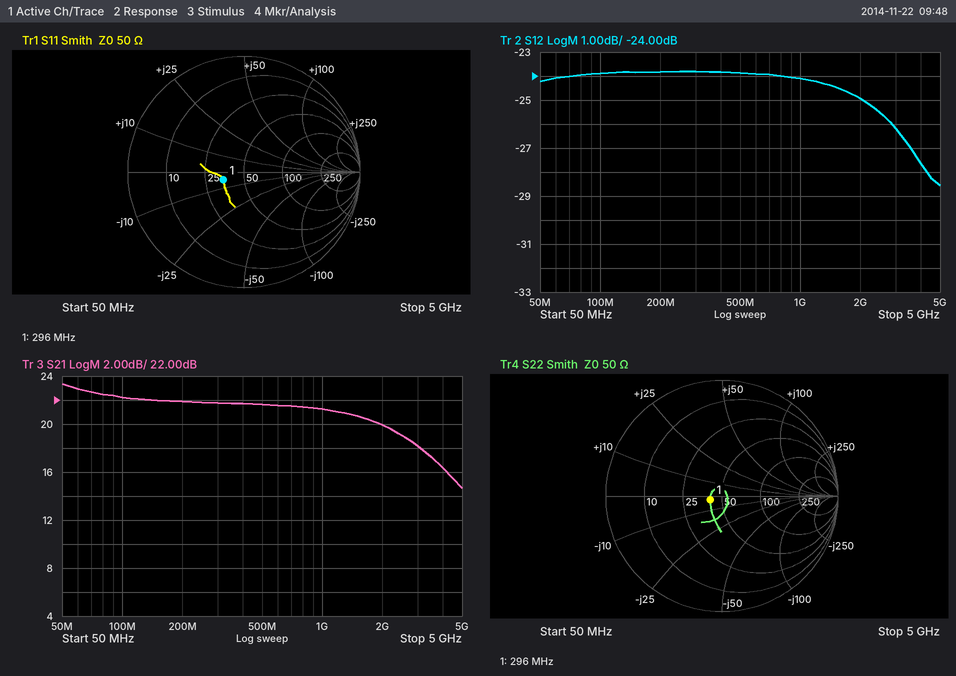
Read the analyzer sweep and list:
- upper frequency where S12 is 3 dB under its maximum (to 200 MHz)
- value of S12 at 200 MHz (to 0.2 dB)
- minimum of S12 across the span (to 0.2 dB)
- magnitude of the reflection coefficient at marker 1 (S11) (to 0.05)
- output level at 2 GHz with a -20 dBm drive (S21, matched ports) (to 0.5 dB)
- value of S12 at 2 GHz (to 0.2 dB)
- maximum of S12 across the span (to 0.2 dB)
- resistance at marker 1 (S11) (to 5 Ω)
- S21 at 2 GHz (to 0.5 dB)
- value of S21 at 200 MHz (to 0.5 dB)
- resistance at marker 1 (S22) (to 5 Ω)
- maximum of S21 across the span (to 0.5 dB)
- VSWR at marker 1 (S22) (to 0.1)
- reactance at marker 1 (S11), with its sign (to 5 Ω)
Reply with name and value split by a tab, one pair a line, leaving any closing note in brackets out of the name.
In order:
upper frequency where S12 is 3 dB under its maximum	3.4 GHz
value of S12 at 200 MHz	-23.8 dB
minimum of S12 across the span	-28.6 dB
magnitude of the reflection coefficient at marker 1 (S11)	0.20
output level at 2 GHz with a -20 dBm drive (S21, matched ports)	0.0 dBm
value of S12 at 2 GHz	-25.0 dB
maximum of S12 across the span	-23.8 dB
resistance at marker 1 (S11)	35 Ω
S21 at 2 GHz	20.0 dB
value of S21 at 200 MHz	22.0 dB
resistance at marker 1 (S22)	40 Ω
maximum of S21 across the span	23.5 dB
VSWR at marker 1 (S22)	1.2
reactance at marker 1 (S11), with its sign	-5 Ω
